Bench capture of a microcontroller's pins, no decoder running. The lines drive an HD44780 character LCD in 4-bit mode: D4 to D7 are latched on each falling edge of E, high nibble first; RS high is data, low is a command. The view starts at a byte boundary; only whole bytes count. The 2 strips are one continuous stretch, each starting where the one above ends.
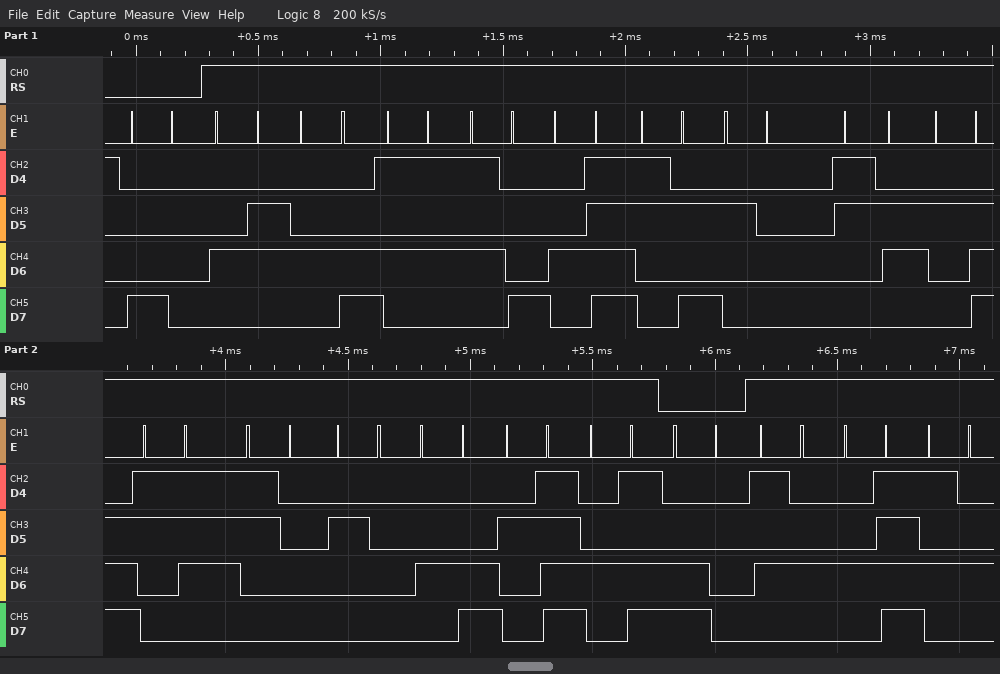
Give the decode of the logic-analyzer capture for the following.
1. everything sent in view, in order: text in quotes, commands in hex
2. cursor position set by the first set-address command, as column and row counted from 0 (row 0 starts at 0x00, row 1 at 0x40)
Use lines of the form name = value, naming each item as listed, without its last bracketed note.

everything sent in view, in order: text in quotes, commands in hex = 0x80 "FLUXO: 6.70 L/M" 0xC0 "TOT"
cursor position set by the first set-address command, as column and row counted from 0 = column 0, row 0
